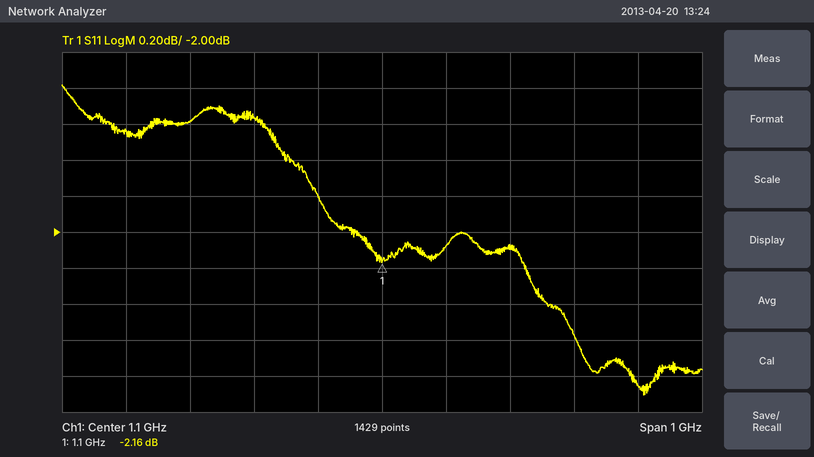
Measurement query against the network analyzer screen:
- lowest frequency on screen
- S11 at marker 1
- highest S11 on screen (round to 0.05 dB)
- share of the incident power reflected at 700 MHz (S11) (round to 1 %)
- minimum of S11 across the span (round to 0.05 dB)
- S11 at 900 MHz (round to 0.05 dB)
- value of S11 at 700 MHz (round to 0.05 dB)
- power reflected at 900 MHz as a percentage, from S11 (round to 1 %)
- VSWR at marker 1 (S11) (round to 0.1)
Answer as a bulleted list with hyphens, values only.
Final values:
- 600 MHz
- -2.16 dB
- -1.20 dB
- 72 %
- -2.90 dB
- -1.35 dB
- -1.45 dB
- 73 %
- 8.1
